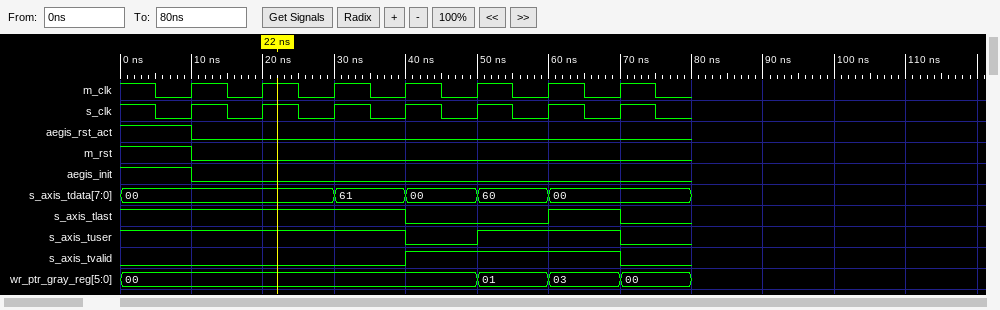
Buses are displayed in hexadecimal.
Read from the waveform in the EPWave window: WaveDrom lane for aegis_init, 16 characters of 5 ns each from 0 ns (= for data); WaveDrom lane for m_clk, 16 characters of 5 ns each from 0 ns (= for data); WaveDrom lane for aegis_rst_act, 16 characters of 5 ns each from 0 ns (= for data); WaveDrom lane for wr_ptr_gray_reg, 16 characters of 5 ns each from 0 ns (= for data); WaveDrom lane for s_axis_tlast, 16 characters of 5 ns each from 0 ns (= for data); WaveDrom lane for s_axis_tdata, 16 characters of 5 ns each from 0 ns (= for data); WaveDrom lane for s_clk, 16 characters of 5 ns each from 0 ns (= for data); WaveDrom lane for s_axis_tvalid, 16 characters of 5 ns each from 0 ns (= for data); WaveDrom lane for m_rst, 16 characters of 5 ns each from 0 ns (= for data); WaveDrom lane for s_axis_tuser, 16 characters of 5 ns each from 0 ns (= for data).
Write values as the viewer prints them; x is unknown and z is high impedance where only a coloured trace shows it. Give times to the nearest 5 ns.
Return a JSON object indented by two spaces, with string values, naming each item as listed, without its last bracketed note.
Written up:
{
  "WaveDrom lane for aegis_init, 16 characters of 5 ns each from 0 ns": "{name: 'aegis_init', wave: '1.0.............'}",
  "WaveDrom lane for m_clk, 16 characters of 5 ns each from 0 ns": "{name: 'm_clk', wave: '1010101010101010'}",
  "WaveDrom lane for aegis_rst_act, 16 characters of 5 ns each from 0 ns": "{name: 'aegis_rst_act', wave: '1.0.............'}",
  "WaveDrom lane for wr_ptr_gray_reg, 16 characters of 5 ns each from 0 ns": "{name: 'wr_ptr_gray_reg', wave: '=.........=.=.=.', data: '00 01 03 00'}",
  "WaveDrom lane for s_axis_tlast, 16 characters of 5 ns each from 0 ns": "{name: 's_axis_tlast', wave: '1.......0...1.0.'}",
  "WaveDrom lane for s_axis_tdata, 16 characters of 5 ns each from 0 ns": "{name: 's_axis_tdata', wave: '=.....=.=.=.=...', data: '00 61 00 60 00'}",
  "WaveDrom lane for s_clk, 16 characters of 5 ns each from 0 ns": "{name: 's_clk', wave: '1010101010101010'}",
  "WaveDrom lane for s_axis_tvalid, 16 characters of 5 ns each from 0 ns": "{name: 's_axis_tvalid', wave: '0.......1.....0.'}",
  "WaveDrom lane for m_rst, 16 characters of 5 ns each from 0 ns": "{name: 'm_rst', wave: '1.0.............'}",
  "WaveDrom lane for s_axis_tuser, 16 characters of 5 ns each from 0 ns": "{name: 's_axis_tuser', wave: '1.......0.1...0.'}"
}
